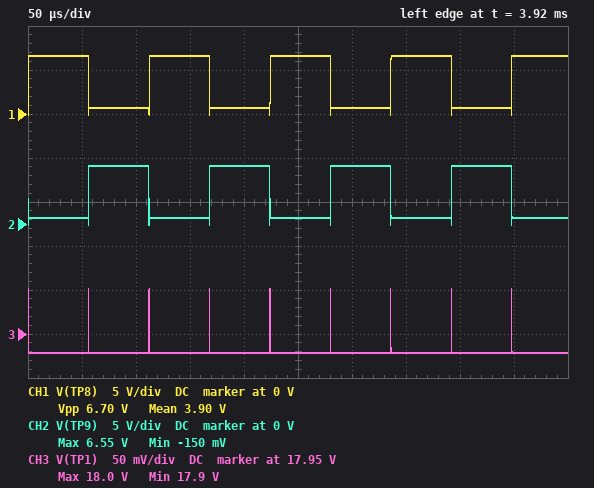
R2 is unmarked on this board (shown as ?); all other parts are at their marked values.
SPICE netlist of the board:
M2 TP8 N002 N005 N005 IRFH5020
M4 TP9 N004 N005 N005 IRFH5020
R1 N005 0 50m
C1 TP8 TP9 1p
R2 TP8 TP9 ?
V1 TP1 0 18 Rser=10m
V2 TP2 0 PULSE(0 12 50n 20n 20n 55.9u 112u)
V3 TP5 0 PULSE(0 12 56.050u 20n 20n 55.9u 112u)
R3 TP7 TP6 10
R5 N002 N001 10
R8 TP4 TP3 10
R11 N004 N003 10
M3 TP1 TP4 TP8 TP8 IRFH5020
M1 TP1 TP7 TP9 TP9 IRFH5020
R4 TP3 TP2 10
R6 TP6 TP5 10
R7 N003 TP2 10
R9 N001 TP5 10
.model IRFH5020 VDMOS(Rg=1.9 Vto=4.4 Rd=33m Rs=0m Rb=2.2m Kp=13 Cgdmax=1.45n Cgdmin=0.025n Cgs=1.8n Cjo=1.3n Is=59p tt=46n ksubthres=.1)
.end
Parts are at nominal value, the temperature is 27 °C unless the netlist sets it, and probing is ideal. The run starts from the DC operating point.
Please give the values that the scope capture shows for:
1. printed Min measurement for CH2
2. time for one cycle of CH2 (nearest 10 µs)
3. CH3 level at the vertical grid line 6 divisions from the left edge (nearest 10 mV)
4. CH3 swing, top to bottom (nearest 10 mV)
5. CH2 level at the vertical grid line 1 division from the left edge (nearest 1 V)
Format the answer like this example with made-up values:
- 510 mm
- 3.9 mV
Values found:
- -150 mV
- 110 µs
- 17.93 V
- 70 mV
- 1 V
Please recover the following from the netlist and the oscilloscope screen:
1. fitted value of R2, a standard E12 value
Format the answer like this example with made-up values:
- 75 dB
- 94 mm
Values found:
- 0.82 Ω
